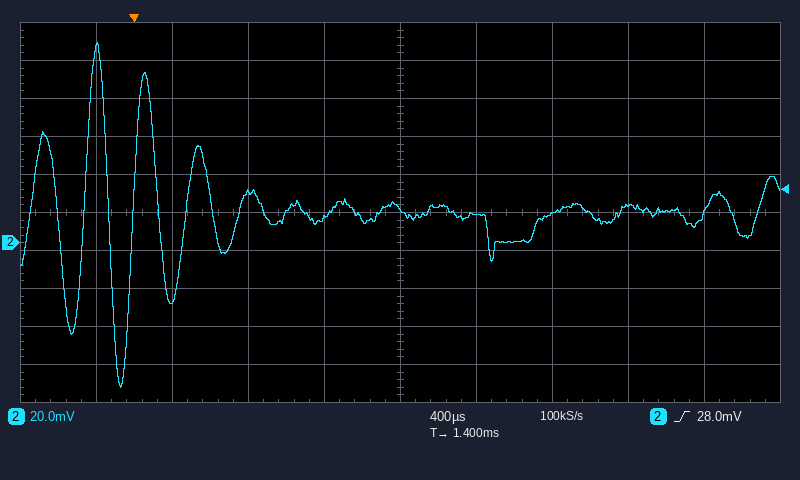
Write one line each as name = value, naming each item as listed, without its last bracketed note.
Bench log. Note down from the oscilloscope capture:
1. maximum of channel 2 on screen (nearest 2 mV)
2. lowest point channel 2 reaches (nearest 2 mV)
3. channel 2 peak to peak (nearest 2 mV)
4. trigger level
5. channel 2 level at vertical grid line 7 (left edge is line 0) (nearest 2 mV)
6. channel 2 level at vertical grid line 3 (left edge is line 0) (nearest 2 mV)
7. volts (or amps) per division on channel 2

maximum of channel 2 on screen = 106 mV
lowest point channel 2 reaches = -76 mV
channel 2 peak to peak = 182 mV
trigger level = 28.0 mV
channel 2 level at vertical grid line 7 (left edge is line 0) = 16 mV
channel 2 level at vertical grid line 3 (left edge is line 0) = 26 mV
volts (or amps) per division on channel 2 = 20 mV
